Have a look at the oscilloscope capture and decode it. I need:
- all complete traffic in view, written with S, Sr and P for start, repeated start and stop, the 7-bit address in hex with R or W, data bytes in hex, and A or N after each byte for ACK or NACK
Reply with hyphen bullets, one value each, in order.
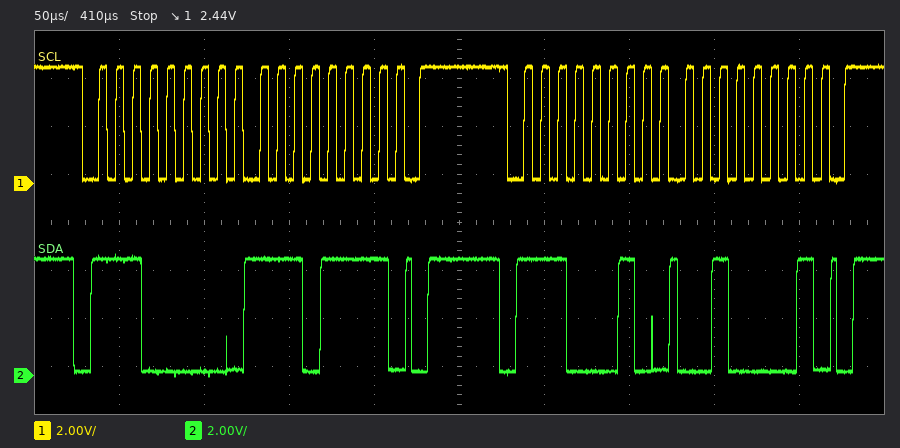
- S 70W A EF A P S 71W A 21 A P
